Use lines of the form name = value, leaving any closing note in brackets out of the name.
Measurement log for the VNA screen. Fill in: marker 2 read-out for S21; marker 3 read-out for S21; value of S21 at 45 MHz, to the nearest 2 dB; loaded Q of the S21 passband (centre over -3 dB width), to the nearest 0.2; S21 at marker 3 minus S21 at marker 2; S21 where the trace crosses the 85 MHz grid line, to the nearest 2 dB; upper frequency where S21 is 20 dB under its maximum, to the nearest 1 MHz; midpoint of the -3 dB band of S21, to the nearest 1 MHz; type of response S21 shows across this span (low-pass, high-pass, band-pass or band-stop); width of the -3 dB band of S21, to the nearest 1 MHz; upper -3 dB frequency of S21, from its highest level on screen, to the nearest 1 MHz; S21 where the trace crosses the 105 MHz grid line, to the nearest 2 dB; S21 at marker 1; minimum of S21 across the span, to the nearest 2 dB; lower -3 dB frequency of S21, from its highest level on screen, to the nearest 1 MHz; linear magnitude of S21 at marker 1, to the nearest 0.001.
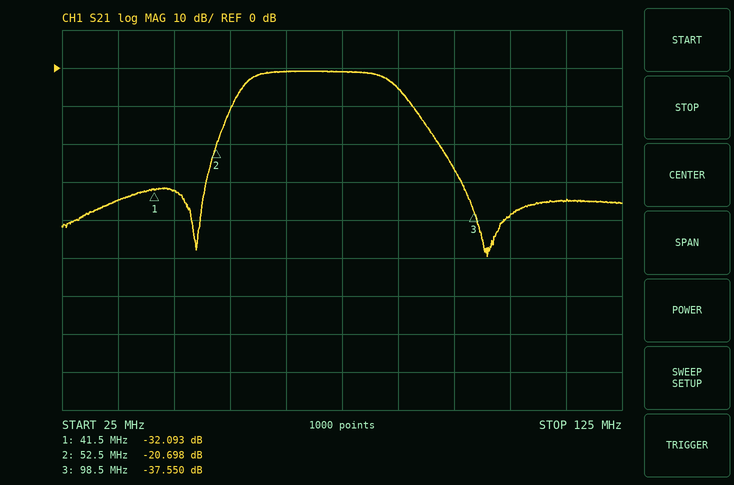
marker 2 read-out for S21 = -20.698 dB
marker 3 read-out for S21 = -37.550 dB
value of S21 at 45 MHz, to the nearest 2 dB = -32 dB
loaded Q of the S21 passband (centre over -3 dB width), to the nearest 0.2 = 2.8
S21 at marker 3 minus S21 at marker 2 = -16.852 dB
S21 where the trace crosses the 85 MHz grid line, to the nearest 2 dB = -6 dB
upper frequency where S21 is 20 dB under its maximum, to the nearest 1 MHz = 93 MHz
midpoint of the -3 dB band of S21, to the nearest 1 MHz = 71 MHz
type of response S21 shows across this span = band-pass
width of the -3 dB band of S21, to the nearest 1 MHz = 26 MHz
upper -3 dB frequency of S21, from its highest level on screen, to the nearest 1 MHz = 84 MHz
S21 where the trace crosses the 105 MHz grid line, to the nearest 2 dB = -38 dB
S21 at marker 1 = -32.093 dB
minimum of S21 across the span, to the nearest 2 dB = -50 dB
lower -3 dB frequency of S21, from its highest level on screen, to the nearest 1 MHz = 58 MHz
linear magnitude of S21 at marker 1, to the nearest 0.001 = 0.025
